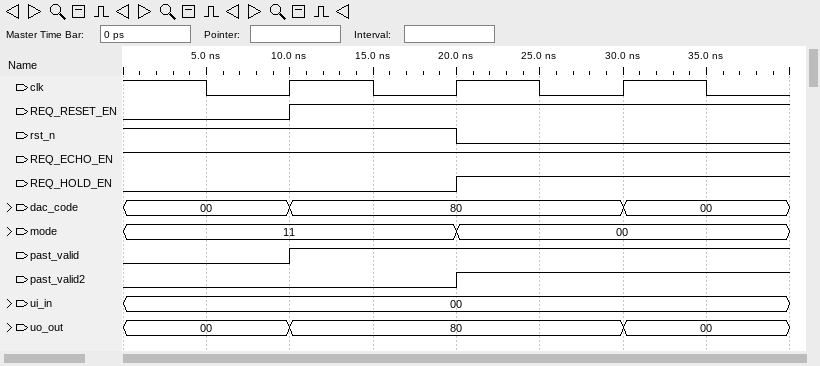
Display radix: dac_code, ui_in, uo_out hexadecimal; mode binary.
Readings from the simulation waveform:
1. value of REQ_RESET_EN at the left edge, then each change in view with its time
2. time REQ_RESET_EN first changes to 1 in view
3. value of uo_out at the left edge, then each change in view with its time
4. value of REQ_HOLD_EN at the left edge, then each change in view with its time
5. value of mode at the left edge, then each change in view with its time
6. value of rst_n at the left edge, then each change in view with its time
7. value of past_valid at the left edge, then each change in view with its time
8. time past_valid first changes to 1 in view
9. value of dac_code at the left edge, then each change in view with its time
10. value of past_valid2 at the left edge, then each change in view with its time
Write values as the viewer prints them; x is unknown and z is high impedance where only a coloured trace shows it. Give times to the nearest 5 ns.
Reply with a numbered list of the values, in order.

1. 0, 1 at 10 ns
2. 10 ns
3. 00, 80 at 10 ns, 00 at 30 ns
4. 0, 1 at 20 ns
5. 11, 00 at 20 ns
6. 1, 0 at 20 ns
7. 0, 1 at 10 ns
8. 10 ns
9. 00, 80 at 10 ns, 00 at 30 ns
10. 0, 1 at 20 ns
